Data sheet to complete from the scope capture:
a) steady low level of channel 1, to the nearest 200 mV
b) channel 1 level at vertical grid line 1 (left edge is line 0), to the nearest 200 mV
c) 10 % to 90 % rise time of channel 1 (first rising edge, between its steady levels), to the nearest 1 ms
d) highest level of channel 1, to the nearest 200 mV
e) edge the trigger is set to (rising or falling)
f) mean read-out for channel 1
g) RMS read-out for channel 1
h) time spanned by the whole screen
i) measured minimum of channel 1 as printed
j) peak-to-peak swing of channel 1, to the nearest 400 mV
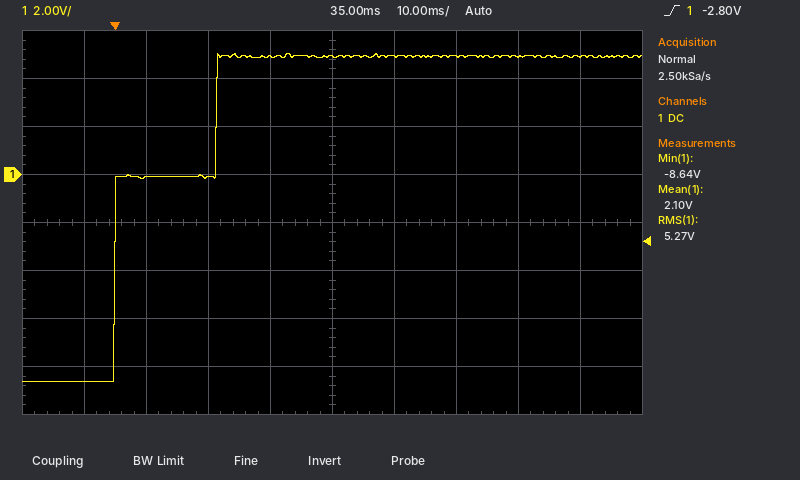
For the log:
-8.6 V
-8.6 V
17 ms
5.0 V
rising
2.10 V
5.27 V
100 ms
-8.64 V
13.6 V
